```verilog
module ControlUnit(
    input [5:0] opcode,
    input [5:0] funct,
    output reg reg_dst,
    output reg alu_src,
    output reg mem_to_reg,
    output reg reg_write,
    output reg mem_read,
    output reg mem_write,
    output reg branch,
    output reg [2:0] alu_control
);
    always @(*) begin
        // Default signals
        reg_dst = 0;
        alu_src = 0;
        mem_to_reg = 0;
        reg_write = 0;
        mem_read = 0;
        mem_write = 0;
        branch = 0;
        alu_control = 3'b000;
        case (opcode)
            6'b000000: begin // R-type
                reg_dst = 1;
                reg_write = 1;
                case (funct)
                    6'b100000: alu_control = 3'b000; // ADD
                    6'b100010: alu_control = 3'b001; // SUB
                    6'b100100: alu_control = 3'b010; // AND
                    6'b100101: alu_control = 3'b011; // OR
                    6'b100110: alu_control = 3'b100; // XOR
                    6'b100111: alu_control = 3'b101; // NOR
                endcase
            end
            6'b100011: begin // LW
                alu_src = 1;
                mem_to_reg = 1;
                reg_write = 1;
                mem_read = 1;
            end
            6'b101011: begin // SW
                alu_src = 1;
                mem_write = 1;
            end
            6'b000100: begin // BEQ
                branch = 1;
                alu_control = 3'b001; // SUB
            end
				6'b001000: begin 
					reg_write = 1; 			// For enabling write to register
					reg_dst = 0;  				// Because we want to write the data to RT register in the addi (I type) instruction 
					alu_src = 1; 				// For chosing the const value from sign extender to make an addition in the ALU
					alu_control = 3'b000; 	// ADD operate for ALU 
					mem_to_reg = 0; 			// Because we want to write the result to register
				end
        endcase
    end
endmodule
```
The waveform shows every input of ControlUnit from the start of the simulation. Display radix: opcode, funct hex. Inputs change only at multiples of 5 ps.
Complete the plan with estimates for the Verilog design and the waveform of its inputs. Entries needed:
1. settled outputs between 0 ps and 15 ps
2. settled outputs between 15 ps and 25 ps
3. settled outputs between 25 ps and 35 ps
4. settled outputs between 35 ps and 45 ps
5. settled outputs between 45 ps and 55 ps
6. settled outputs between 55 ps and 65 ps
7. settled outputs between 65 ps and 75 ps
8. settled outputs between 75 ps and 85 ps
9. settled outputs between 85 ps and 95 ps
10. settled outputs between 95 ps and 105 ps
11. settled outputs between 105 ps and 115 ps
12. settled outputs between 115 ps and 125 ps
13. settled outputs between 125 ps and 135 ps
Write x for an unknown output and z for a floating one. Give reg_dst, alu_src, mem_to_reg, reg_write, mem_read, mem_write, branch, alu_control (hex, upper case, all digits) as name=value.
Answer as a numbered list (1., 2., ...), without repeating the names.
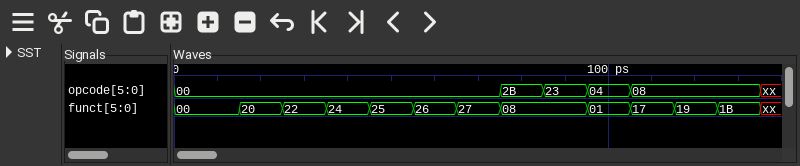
1. reg_dst=1, alu_src=0, mem_to_reg=0, reg_write=1, mem_read=0, mem_write=0, branch=0, alu_control=0
2. reg_dst=1, alu_src=0, mem_to_reg=0, reg_write=1, mem_read=0, mem_write=0, branch=0, alu_control=0
3. reg_dst=1, alu_src=0, mem_to_reg=0, reg_write=1, mem_read=0, mem_write=0, branch=0, alu_control=1
4. reg_dst=1, alu_src=0, mem_to_reg=0, reg_write=1, mem_read=0, mem_write=0, branch=0, alu_control=2
5. reg_dst=1, alu_src=0, mem_to_reg=0, reg_write=1, mem_read=0, mem_write=0, branch=0, alu_control=3
6. reg_dst=1, alu_src=0, mem_to_reg=0, reg_write=1, mem_read=0, mem_write=0, branch=0, alu_control=4
7. reg_dst=1, alu_src=0, mem_to_reg=0, reg_write=1, mem_read=0, mem_write=0, branch=0, alu_control=5
8. reg_dst=0, alu_src=1, mem_to_reg=0, reg_write=0, mem_read=0, mem_write=1, branch=0, alu_control=0
9. reg_dst=0, alu_src=1, mem_to_reg=1, reg_write=1, mem_read=1, mem_write=0, branch=0, alu_control=0
10. reg_dst=0, alu_src=0, mem_to_reg=0, reg_write=0, mem_read=0, mem_write=0, branch=1, alu_control=1
11. reg_dst=0, alu_src=1, mem_to_reg=0, reg_write=1, mem_read=0, mem_write=0, branch=0, alu_control=0
12. reg_dst=0, alu_src=1, mem_to_reg=0, reg_write=1, mem_read=0, mem_write=0, branch=0, alu_control=0
13. reg_dst=0, alu_src=1, mem_to_reg=0, reg_write=1, mem_read=0, mem_write=0, branch=0, alu_control=0
